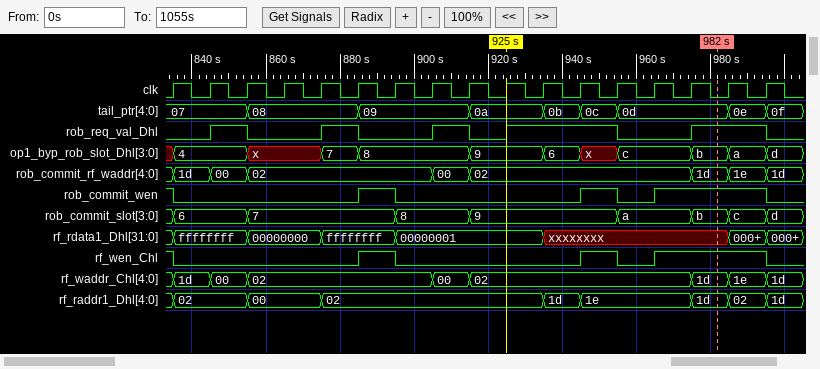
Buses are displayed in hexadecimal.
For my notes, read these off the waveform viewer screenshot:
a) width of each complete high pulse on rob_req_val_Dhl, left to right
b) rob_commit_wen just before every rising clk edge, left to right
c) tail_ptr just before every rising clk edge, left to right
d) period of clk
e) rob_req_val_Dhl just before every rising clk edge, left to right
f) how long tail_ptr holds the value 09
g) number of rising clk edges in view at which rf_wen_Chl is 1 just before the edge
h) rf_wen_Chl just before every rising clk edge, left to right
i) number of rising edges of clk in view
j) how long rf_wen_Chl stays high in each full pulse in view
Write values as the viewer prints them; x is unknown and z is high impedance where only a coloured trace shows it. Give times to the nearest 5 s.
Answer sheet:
10 s, 10 s, 10 s, 30 s, 20 s
1 0 0 0 0 0 1 0 0 0 0 0 1 0 1 1 1
07, 07, 07, 08, 08, 08, 09, 09, 09, 0a, 0a, 0b, 0c, 0d, 0d, 0d, 0e
10 s
0 0 1 0 0 1 0 0 1 0 1 1 1 0 0 1 1
30 s
6
1 0 0 0 0 0 1 0 0 0 0 0 1 0 1 1 1
17
10 s, 10 s, 30 s
